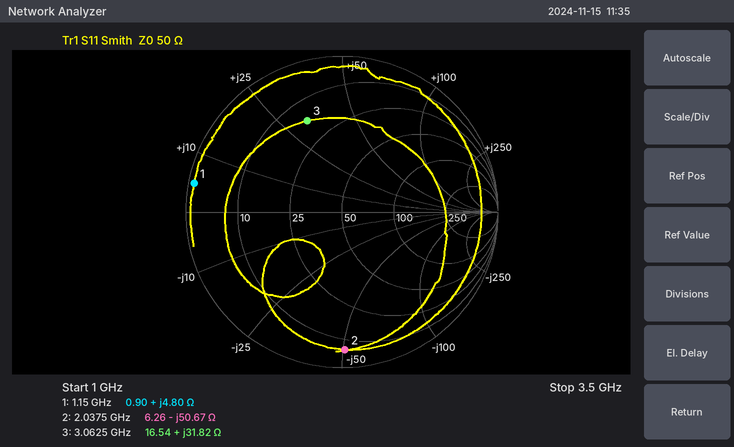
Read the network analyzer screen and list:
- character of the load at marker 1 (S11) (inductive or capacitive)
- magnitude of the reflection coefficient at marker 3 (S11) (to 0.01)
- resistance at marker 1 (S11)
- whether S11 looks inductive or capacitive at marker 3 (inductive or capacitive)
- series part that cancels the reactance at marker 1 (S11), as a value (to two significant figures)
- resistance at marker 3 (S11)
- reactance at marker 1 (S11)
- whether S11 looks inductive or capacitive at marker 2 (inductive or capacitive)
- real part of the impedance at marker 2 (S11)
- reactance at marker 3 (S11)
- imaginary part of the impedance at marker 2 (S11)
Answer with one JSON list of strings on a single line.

["inductive", "0.63", "0.90 Ω", "inductive", "29 pF", "16.54 Ω", "+4.80 Ω", "capacitive", "6.26 Ω", "+31.82 Ω", "-50.67 Ω"]
